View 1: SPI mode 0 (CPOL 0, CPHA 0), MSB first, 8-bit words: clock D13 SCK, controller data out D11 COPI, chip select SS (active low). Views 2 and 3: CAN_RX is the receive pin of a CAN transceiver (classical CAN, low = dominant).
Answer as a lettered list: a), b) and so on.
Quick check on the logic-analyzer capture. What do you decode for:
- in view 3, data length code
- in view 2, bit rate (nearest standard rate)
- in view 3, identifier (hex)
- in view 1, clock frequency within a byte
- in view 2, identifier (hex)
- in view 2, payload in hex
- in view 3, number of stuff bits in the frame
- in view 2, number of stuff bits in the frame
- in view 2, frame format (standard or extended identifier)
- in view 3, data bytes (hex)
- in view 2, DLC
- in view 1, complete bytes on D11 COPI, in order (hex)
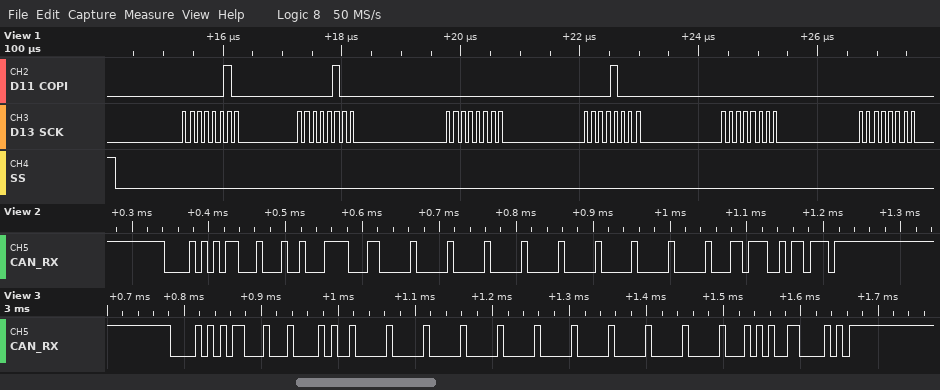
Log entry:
a) 8
b) 125 kbit/s
c) 0x0AB
d) 8 MHz
e) 0x0AB
f) 91 E3 00 00 00 00 00 00
g) 10
h) 9
i) standard
j) 85 20 00 00 00 00 00 00
k) 8
l) 02 04 00 08 00 00
